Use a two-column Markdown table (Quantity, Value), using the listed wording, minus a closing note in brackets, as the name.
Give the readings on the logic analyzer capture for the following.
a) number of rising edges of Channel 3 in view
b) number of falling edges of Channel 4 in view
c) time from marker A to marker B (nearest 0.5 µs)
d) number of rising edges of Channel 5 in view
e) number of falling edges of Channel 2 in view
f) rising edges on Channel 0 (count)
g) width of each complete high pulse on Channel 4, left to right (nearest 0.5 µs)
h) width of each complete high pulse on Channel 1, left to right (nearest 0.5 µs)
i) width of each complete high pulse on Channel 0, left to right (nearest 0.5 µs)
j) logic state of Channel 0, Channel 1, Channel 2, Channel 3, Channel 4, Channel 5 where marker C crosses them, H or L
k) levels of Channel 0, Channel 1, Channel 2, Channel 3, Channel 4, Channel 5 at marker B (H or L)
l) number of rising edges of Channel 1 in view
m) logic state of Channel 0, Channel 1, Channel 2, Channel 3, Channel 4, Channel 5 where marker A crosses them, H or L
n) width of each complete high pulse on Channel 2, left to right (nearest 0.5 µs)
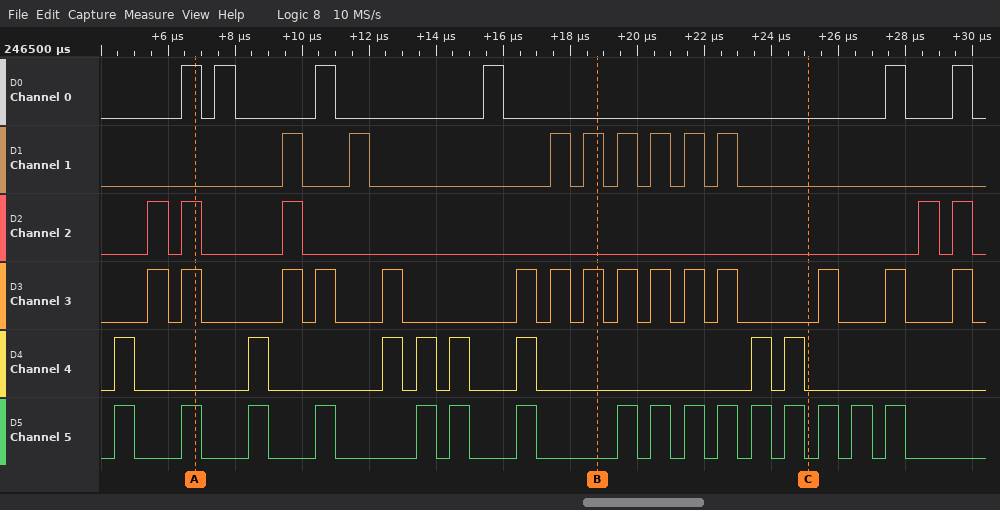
| Quantity | Value |
|---|---|
| number of rising edges of Channel 3 in view | 15 |
| number of falling edges of Channel 4 in view | 8 |
| time from marker A to marker B | 12 µs |
| number of rising edges of Channel 5 in view | 16 |
| number of falling edges of Channel 2 in view | 5 |
| rising edges on Channel 0 | 6 |
| width of each complete high pulse on Channel 4, left to right | 0.5 µs, 0.5 µs, 0.5 µs, 0.5 µs, 0.5 µs, 0.5 µs, 0.5 µs, 0.5 µs |
| width of each complete high pulse on Channel 1, left to right | 0.5 µs, 0.5 µs, 0.5 µs, 0.5 µs, 0.5 µs, 0.5 µs, 0.5 µs, 0.5 µs |
| width of each complete high pulse on Channel 0, left to right | 0.5 µs, 0.5 µs, 0.5 µs, 0.5 µs, 0.5 µs, 0.5 µs |
| logic state of Channel 0, Channel 1, Channel 2, Channel 3, Channel 4, Channel 5 where marker C crosses them, H or L | Channel 0=L, Channel 1=L, Channel 2=L, Channel 3=L, Channel 4=L, Channel 5=L |
| levels of Channel 0, Channel 1, Channel 2, Channel 3, Channel 4, Channel 5 at marker B | Channel 0=L, Channel 1=H, Channel 2=L, Channel 3=H, Channel 4=L, Channel 5=L |
| number of rising edges of Channel 1 in view | 8 |
| logic state of Channel 0, Channel 1, Channel 2, Channel 3, Channel 4, Channel 5 where marker A crosses them, H or L | Channel 0=H, Channel 1=L, Channel 2=H, Channel 3=H, Channel 4=L, Channel 5=H |
| width of each complete high pulse on Channel 2, left to right | 0.5 µs, 0.5 µs, 0.5 µs, 0.5 µs, 0.5 µs |
